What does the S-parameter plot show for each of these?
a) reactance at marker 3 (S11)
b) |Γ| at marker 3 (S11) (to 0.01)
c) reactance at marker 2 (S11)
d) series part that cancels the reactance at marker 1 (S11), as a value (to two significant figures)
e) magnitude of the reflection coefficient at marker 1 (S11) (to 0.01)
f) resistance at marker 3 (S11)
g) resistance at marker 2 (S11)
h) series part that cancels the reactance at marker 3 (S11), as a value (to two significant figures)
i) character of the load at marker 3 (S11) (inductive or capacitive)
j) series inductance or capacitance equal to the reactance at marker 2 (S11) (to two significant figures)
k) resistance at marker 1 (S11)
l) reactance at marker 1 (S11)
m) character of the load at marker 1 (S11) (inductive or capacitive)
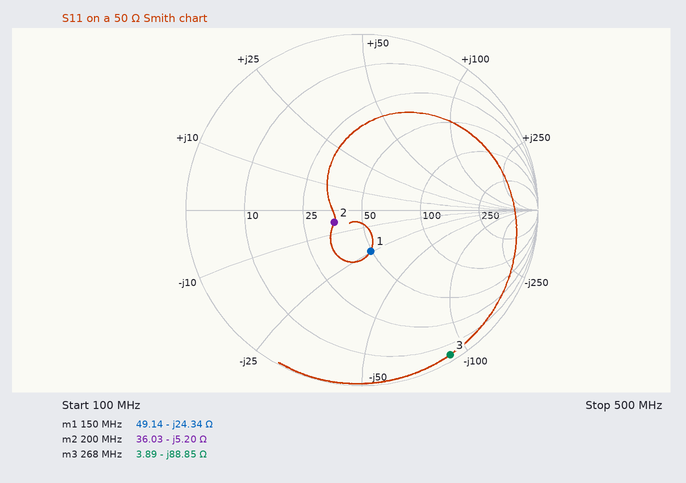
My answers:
-88.85 Ω
0.96
-5.20 Ω
26 nH
0.24
3.89 Ω
36.03 Ω
53 nH
capacitive
150 pF
49.14 Ω
-24.34 Ω
capacitive
